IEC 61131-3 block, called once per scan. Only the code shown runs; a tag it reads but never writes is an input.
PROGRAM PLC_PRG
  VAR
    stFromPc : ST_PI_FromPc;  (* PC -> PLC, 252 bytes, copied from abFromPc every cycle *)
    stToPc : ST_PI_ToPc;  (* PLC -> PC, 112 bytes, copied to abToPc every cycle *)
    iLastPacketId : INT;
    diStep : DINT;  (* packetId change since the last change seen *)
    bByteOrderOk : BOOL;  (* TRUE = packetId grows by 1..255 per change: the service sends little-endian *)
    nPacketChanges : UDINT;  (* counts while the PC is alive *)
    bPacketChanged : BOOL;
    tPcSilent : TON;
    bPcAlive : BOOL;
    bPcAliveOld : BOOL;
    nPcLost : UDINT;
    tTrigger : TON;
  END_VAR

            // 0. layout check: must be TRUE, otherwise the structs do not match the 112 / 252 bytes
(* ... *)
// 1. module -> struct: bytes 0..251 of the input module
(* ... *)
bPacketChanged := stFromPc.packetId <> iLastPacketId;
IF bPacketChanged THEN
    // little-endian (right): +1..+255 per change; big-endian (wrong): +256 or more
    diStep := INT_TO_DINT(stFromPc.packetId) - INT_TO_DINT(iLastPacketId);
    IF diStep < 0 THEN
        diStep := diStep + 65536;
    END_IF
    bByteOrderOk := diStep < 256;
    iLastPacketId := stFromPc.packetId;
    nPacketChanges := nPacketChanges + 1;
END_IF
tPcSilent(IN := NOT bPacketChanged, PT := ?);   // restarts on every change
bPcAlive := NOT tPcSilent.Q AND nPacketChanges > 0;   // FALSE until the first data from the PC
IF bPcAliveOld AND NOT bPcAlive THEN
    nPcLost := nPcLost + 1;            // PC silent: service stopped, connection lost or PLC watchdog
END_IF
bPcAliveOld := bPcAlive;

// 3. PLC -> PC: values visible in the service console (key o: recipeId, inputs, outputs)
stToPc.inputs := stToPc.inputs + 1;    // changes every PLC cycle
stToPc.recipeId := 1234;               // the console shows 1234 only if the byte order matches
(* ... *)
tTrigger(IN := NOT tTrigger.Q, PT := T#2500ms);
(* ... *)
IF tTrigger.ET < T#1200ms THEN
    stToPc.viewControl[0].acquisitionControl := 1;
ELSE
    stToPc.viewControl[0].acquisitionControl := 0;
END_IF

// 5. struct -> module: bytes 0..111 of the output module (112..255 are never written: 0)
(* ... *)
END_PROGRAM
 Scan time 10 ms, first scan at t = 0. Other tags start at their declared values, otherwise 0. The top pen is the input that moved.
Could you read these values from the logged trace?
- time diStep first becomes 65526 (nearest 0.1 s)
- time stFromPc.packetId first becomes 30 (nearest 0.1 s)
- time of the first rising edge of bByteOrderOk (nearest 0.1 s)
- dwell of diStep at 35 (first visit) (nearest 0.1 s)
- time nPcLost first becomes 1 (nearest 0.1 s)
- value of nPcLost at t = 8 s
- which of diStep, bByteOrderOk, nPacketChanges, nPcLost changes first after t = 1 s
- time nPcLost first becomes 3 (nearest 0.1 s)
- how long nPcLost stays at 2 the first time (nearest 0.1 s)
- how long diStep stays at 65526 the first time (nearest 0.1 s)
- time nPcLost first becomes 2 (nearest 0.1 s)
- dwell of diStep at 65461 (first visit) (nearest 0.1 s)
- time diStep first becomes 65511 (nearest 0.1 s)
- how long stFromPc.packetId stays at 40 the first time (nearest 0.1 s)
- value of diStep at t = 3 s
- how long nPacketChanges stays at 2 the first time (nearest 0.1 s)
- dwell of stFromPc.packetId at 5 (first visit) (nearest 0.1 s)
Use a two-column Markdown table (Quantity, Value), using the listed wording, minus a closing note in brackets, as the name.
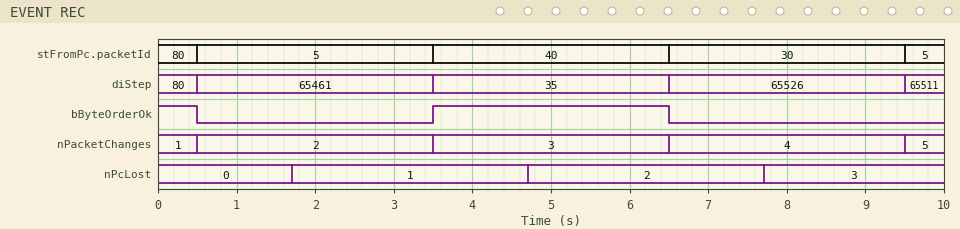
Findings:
| Quantity | Value |
|---|---|
| time diStep first becomes 65526 | 6.5 s |
| time stFromPc.packetId first becomes 30 | 6.5 s |
| time of the first rising edge of bByteOrderOk | 3.5 s |
| dwell of diStep at 35 (first visit) | 3.0 s |
| time nPcLost first becomes 1 | 1.7 s |
| value of nPcLost at t = 8 s | 3 |
| which of diStep, bByteOrderOk, nPacketChanges, nPcLost changes first after t = 1 s | nPcLost |
| time nPcLost first becomes 3 | 7.7 s |
| how long nPcLost stays at 2 the first time | 3.0 s |
| how long diStep stays at 65526 the first time | 3.0 s |
| time nPcLost first becomes 2 | 4.7 s |
| dwell of diStep at 65461 (first visit) | 3.0 s |
| time diStep first becomes 65511 | 9.5 s |
| how long stFromPc.packetId stays at 40 the first time | 3.0 s |
| value of diStep at t = 3 s | 65461 |
| how long nPacketChanges stays at 2 the first time | 3.0 s |
| dwell of stFromPc.packetId at 5 (first visit) | 3.0 s |
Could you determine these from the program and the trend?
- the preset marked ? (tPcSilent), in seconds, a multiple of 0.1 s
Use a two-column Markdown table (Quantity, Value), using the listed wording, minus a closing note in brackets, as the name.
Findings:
| Quantity | Value |
|---|---|
| the preset marked ? (tPcSilent), in seconds, a multiple of 0.1 s | 1.2 s |
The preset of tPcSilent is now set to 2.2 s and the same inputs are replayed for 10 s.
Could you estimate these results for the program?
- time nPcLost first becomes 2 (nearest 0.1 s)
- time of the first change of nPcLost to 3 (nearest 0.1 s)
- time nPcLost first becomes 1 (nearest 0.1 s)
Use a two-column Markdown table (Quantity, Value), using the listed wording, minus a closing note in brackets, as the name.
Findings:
| Quantity | Value |
|---|---|
| time nPcLost first becomes 2 | 5.7 s |
| time of the first change of nPcLost to 3 | 8.7 s |
| time nPcLost first becomes 1 | 2.7 s |
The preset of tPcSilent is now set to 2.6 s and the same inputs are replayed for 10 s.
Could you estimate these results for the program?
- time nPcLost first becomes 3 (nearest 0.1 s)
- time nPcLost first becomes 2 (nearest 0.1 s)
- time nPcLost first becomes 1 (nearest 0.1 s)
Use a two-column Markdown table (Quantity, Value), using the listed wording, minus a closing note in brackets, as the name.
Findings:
| Quantity | Value |
|---|---|
| time nPcLost first becomes 3 | 9.1 s |
| time nPcLost first becomes 2 | 6.1 s |
| time nPcLost first becomes 1 | 3.1 s |
